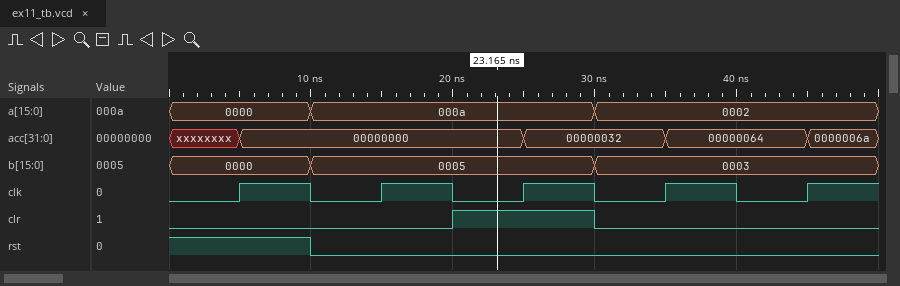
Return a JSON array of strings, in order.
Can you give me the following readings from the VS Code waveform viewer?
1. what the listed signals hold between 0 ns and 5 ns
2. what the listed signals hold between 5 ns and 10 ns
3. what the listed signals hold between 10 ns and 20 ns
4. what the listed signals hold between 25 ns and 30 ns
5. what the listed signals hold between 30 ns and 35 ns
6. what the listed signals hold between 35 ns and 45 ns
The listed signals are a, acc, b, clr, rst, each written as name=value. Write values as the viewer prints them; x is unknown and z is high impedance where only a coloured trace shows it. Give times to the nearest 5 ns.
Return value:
["a=0000, acc=xxxxxxxx, b=0000, clr=0, rst=1", "a=0000, acc=00000000, b=0000, clr=0, rst=1", "a=000a, acc=00000000, b=0005, clr=0, rst=0", "a=000a, acc=00000032, b=0005, clr=1, rst=0", "a=0002, acc=00000032, b=0003, clr=0, rst=0", "a=0002, acc=00000064, b=0003, clr=0, rst=0"]
